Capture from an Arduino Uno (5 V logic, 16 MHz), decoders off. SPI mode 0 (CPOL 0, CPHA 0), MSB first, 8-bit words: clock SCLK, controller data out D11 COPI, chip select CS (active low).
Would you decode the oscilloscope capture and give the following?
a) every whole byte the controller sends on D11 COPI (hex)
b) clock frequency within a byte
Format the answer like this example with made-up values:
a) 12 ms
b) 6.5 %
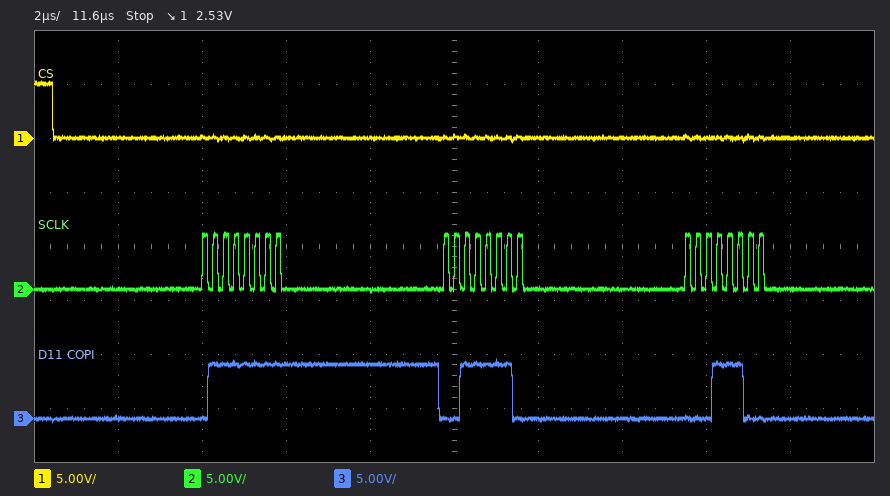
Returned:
a) 0x7F 0x3E 0x1C
b) 4 MHz
